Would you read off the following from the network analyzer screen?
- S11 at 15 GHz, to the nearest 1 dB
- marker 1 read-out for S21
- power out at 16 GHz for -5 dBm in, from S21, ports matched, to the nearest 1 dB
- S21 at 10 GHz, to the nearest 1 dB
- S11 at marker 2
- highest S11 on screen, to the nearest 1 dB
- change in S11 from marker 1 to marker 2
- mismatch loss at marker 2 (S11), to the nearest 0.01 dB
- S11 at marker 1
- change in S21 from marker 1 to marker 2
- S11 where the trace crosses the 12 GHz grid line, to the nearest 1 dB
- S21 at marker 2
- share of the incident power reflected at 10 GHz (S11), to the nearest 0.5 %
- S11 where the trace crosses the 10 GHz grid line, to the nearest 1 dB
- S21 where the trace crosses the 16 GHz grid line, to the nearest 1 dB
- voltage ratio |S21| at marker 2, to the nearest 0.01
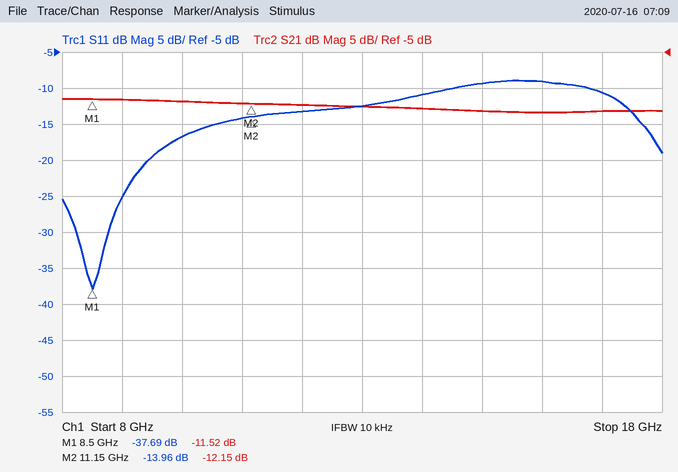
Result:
-9 dB
-11.52 dB
-18 dBm
-12 dB
-13.96 dB
-9 dB
23.73 dB
0.18 dB
-37.69 dB
-0.63 dB
-13 dB
-12.15 dB
2.0 %
-17 dB
-13 dB
0.25
